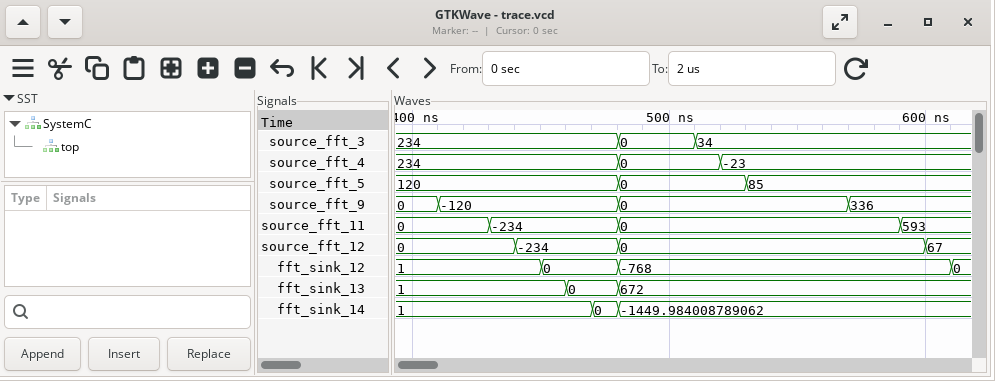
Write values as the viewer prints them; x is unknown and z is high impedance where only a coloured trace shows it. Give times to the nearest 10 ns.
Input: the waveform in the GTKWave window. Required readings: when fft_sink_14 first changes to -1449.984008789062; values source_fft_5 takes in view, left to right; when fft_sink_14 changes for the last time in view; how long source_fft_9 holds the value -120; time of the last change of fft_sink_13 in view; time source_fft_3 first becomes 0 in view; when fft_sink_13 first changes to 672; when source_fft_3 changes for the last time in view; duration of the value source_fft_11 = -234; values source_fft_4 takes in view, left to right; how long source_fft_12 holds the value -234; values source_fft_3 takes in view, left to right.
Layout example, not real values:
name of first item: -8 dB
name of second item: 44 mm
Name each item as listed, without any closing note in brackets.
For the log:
when fft_sink_14 first changes to -1449.984008789062: 480 ns
values source_fft_5 takes in view, left to right: 120, 0, 85
when fft_sink_14 changes for the last time in view: 480 ns
how long source_fft_9 holds the value -120: 70 ns
time of the last change of fft_sink_13 in view: 480 ns
time source_fft_3 first becomes 0 in view: 480 ns
when fft_sink_13 first changes to 672: 480 ns
when source_fft_3 changes for the last time in view: 510 ns
duration of the value source_fft_11 = -234: 50 ns
values source_fft_4 takes in view, left to right: 234, 0, -23
how long source_fft_12 holds the value -234: 40 ns
values source_fft_3 takes in view, left to right: 234, 0, 34
